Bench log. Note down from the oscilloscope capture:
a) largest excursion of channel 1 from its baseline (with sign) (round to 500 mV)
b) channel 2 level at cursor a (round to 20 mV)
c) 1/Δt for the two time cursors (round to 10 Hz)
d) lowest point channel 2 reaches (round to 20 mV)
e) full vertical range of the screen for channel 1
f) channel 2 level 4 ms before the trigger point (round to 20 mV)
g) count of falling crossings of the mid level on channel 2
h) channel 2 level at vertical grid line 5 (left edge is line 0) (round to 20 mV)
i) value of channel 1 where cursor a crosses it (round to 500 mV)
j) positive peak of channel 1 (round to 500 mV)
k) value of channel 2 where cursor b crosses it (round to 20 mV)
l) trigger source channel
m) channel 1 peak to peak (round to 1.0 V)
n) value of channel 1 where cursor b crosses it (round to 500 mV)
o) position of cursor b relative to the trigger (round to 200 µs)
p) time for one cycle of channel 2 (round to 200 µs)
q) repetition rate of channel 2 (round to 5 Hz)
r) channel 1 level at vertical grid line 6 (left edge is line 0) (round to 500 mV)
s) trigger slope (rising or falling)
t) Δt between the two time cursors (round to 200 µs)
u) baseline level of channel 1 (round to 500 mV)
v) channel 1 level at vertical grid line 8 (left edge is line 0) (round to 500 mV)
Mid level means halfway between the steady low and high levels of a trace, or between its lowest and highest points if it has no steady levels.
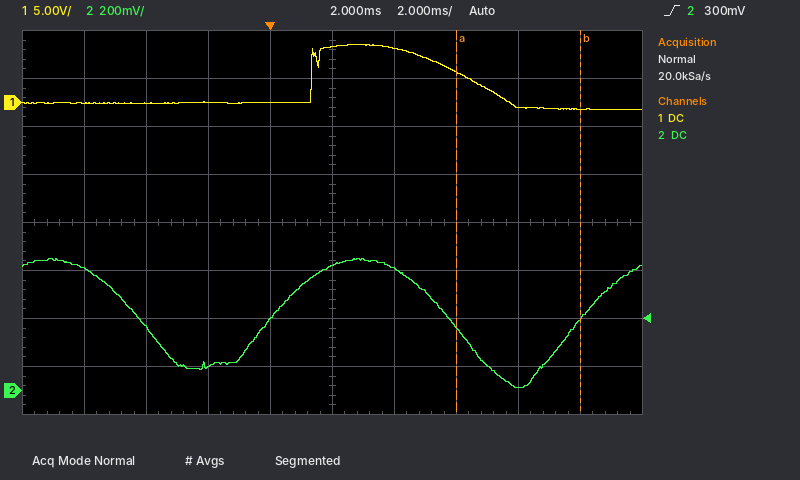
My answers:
+6.0 V
260 mV
250 Hz
20 mV
40 V
260 mV
2
520 mV
3.0 V
6.0 V
300 mV
channel 2
7.0 V
-500 mV
+10.0 ms
10.0 ms
100 Hz
5.5 V
rising
4.0 ms
0.0 V
-500 mV
